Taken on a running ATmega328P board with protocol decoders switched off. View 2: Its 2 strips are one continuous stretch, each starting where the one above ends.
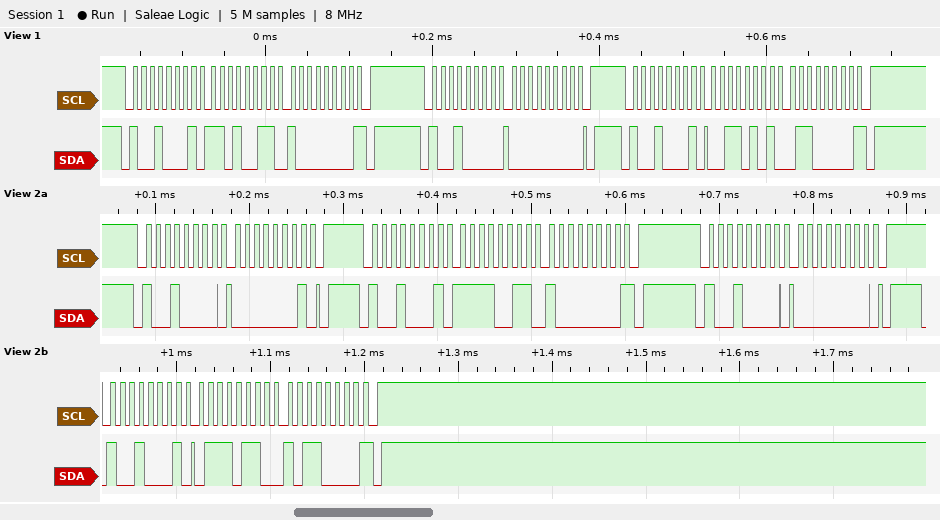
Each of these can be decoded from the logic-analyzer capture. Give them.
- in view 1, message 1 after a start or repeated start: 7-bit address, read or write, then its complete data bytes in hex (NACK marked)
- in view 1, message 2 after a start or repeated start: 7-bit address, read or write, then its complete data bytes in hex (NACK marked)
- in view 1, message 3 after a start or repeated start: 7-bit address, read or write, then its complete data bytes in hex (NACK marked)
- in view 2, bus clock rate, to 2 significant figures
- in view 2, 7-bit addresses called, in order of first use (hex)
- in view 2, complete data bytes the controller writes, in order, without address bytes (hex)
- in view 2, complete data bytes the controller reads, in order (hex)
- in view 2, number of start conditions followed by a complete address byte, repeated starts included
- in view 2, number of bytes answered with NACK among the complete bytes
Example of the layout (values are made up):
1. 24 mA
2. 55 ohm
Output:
1. 0x48 read: D3 80 NACK
2. 0x48 write: 00
3. 0x48 read: 35 60 NACK
4. 100 kHz
5. 0x48
6. 01 00
7. F3 80 76 B0
8. 4
9. 2
